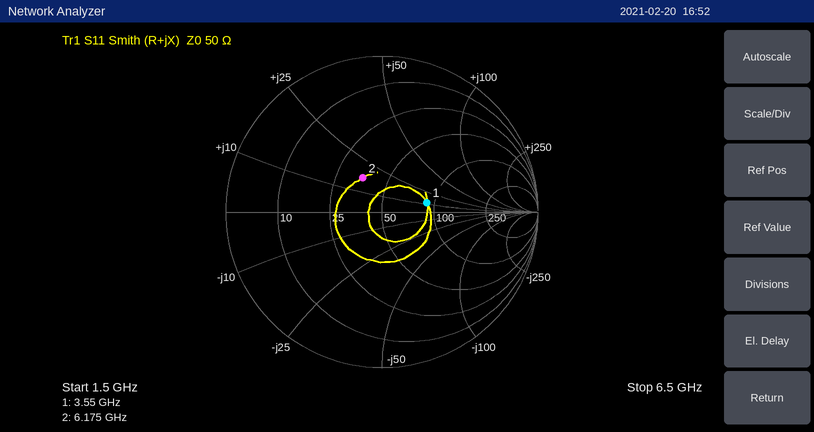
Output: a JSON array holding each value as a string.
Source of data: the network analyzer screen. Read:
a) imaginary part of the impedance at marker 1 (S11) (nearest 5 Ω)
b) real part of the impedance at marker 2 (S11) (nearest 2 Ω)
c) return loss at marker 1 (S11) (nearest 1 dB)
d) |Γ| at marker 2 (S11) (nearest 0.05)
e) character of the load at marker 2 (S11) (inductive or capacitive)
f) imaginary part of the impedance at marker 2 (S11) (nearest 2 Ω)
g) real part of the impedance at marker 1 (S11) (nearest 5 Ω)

["+10 Ω", "36 Ω", "11 dB", "0.25", "inductive", "+16 Ω", "90 Ω"]
